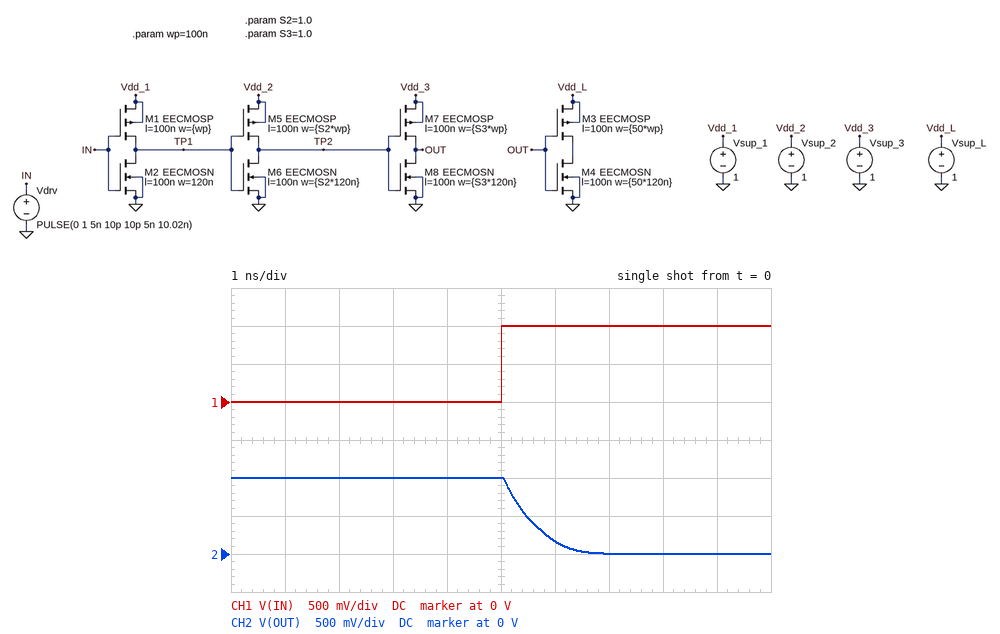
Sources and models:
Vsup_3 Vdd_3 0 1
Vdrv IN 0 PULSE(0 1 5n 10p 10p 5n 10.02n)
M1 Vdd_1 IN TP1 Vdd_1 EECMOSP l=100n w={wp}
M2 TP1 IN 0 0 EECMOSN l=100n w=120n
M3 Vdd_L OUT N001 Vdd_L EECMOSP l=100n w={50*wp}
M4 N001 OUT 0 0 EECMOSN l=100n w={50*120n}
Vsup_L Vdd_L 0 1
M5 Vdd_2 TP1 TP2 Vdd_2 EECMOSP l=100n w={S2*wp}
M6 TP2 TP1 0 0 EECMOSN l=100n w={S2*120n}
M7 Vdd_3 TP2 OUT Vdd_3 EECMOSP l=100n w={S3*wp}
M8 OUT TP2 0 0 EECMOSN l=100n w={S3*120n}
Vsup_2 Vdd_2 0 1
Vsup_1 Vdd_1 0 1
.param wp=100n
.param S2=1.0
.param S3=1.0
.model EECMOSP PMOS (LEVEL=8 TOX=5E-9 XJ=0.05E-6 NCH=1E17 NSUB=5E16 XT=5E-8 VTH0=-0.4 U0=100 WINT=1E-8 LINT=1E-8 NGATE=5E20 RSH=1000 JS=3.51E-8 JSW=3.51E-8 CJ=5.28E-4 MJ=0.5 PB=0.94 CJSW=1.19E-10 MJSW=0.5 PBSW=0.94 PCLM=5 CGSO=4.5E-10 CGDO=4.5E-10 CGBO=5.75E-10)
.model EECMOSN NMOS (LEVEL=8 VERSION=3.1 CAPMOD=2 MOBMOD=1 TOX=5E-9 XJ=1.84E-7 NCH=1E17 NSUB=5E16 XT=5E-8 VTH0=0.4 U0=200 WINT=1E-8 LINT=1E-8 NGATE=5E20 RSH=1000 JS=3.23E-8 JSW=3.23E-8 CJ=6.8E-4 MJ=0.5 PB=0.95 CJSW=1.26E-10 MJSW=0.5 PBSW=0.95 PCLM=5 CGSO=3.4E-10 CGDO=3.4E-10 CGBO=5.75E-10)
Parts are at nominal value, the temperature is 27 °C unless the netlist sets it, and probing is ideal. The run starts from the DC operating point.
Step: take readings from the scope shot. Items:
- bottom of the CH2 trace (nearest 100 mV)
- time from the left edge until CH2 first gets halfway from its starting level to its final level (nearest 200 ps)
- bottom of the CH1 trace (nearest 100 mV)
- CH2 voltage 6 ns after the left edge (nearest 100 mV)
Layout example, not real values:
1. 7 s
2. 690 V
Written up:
1. 0 V
2. 5.4 ns
3. 0 V
4. 200 mV
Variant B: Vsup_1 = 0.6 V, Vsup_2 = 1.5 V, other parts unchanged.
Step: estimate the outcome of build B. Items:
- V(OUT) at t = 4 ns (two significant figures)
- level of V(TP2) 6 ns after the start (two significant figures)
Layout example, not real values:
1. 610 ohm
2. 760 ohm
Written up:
1. 43 mV
2. 1.5 V
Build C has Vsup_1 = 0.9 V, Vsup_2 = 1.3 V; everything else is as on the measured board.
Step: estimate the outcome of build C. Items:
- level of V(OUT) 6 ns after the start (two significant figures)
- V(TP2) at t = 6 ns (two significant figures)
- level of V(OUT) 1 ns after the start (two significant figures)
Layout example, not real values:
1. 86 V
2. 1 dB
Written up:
1. 63 mV
2. 1.3 V
3. 1.0 V
